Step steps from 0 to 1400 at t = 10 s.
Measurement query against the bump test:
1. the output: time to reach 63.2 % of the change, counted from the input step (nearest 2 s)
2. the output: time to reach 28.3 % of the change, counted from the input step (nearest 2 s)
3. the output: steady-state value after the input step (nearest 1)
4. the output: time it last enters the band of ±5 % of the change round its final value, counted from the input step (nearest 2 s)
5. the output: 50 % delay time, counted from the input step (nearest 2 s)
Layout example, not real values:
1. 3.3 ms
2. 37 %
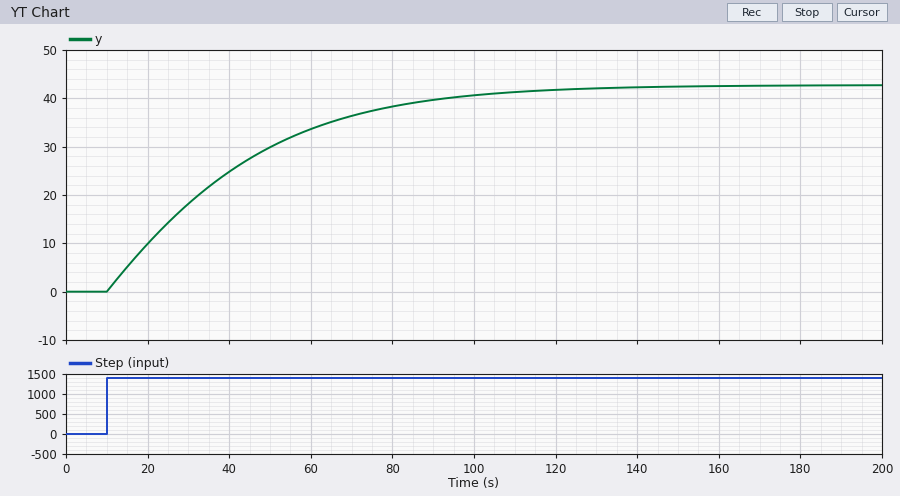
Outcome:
1. 34 s
2. 12 s
3. 43
4. 90 s
5. 24 s
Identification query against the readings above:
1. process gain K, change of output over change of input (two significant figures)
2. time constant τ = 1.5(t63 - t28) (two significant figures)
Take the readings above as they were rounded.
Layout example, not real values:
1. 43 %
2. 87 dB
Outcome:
1. 0.031
2. 33 s
